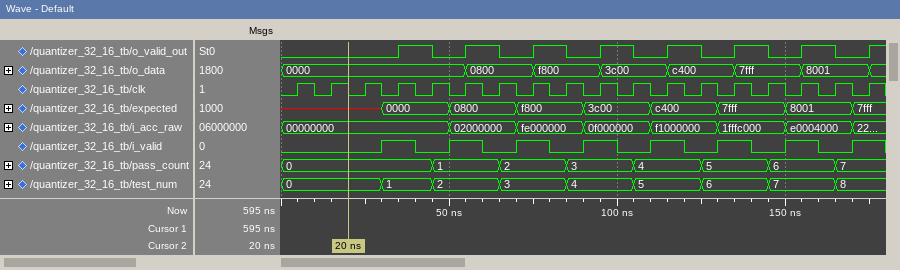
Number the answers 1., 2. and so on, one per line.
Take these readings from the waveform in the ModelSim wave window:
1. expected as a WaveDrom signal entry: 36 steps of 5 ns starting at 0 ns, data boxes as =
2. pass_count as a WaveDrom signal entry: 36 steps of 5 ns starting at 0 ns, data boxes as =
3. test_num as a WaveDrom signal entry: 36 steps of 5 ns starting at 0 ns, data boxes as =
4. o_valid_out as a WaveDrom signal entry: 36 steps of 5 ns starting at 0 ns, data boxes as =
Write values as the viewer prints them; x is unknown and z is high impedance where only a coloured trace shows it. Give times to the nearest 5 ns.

1. {name: 'expected', wave: 'x.....=...=...=...=...=...=...=...=.', data: '0000 0800 f800 3c00 c400 7fff 8001 7fff'}
2. {name: 'pass_count', wave: '=........=...=...=...=...=...=...=..', data: '0 1 2 3 4 5 6 7'}
3. {name: 'test_num', wave: '=.....=..=...=...=...=...=...=...=..', data: '0 1 2 3 4 5 6 7 8'}
4. {name: 'o_valid_out', wave: '0......1.0.1.0.1.0.1.0.1.0.1.0.1.0.1'}
